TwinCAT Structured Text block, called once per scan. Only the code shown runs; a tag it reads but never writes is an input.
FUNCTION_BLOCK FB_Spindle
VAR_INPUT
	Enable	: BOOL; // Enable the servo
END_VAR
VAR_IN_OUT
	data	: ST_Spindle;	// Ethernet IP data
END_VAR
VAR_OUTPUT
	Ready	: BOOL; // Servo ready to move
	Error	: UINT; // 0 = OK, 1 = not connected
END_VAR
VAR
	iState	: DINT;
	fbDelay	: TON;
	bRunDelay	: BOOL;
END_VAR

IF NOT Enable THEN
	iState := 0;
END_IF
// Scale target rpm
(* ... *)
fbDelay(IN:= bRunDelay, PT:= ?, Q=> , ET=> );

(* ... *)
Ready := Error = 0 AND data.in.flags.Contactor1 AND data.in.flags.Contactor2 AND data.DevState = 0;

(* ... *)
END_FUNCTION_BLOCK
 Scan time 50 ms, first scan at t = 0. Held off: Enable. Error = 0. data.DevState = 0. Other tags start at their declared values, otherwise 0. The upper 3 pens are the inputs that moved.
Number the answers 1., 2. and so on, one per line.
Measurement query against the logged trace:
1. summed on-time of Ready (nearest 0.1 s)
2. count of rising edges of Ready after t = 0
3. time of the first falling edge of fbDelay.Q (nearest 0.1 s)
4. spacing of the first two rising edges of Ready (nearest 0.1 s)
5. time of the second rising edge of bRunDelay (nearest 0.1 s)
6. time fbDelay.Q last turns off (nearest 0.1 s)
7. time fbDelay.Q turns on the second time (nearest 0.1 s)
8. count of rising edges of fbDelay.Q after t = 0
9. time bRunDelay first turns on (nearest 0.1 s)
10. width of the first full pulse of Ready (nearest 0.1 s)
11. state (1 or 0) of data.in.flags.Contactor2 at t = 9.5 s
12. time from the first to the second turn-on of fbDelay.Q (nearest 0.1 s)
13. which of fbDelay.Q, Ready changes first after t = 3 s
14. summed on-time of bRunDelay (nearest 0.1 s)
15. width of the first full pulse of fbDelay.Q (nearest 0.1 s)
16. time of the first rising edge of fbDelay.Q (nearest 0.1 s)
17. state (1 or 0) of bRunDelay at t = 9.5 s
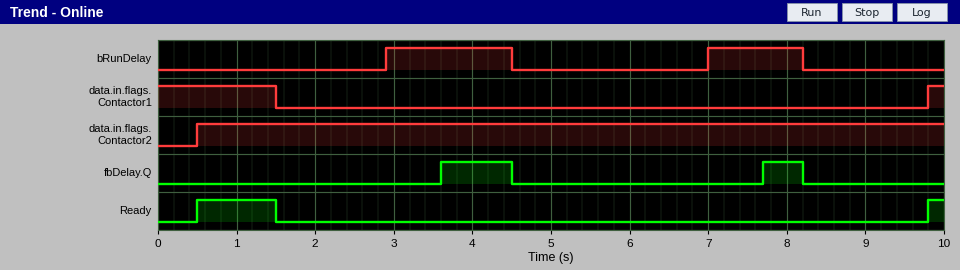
1. 1.2 s
2. 2
3. 4.5 s
4. 9.3 s
5. 7.0 s
6. 8.2 s
7. 7.7 s
8. 2
9. 2.9 s
10. 1.0 s
11. 1
12. 4.1 s
13. fbDelay.Q
14. 2.8 s
15. 0.9 s
16. 3.6 s
17. 0
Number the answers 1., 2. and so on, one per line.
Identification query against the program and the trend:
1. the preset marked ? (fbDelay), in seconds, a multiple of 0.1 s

1. 0.7 s
